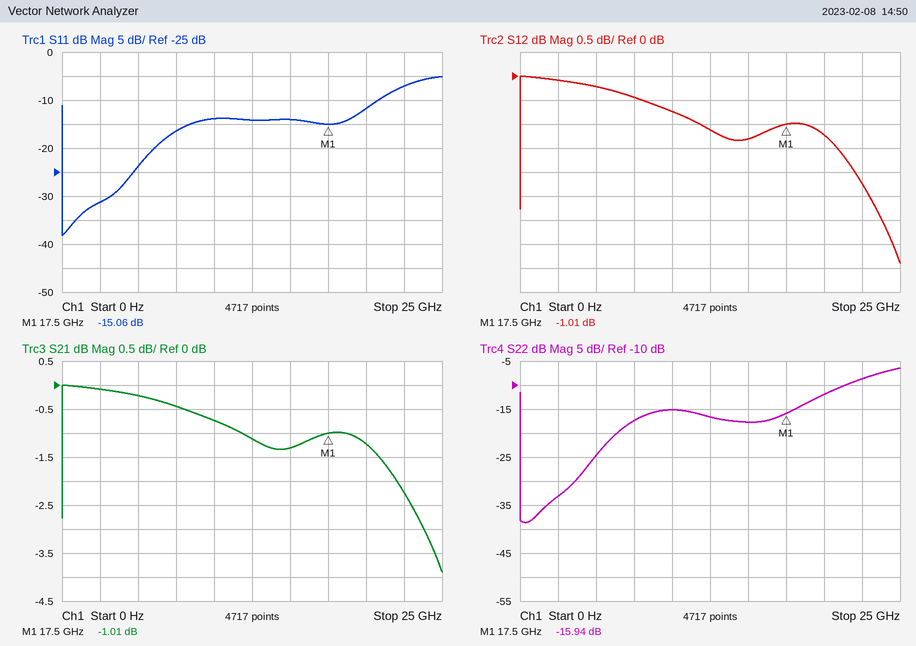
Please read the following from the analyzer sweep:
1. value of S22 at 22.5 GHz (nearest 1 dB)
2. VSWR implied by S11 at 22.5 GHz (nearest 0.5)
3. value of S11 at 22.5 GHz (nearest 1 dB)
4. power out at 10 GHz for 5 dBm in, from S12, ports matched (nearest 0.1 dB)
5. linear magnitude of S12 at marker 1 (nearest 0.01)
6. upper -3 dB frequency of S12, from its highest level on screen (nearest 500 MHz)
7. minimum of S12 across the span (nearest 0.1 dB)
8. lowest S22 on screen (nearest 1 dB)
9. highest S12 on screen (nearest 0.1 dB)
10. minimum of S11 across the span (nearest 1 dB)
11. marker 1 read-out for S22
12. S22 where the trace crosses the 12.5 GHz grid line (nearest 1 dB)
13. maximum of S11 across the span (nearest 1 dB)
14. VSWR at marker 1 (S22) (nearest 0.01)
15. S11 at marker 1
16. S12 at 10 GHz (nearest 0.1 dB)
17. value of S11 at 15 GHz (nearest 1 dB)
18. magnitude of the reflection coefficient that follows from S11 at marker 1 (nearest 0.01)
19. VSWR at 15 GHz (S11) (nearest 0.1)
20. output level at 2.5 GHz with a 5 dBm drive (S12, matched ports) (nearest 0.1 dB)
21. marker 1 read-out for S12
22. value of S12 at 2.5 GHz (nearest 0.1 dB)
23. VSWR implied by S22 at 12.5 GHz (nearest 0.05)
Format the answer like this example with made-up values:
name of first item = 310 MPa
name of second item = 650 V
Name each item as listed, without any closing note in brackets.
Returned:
value of S22 at 22.5 GHz = -9 dB
VSWR implied by S11 at 22.5 GHz = 2.5
value of S11 at 22.5 GHz = -7 dB
power out at 10 GHz for 5 dBm in, from S12, ports matched = 4.3 dBm
linear magnitude of S12 at marker 1 = 0.89
upper -3 dB frequency of S12, from its highest level on screen = 24.0 GHz
minimum of S12 across the span = -3.9 dB
lowest S22 on screen = -39 dB
highest S12 on screen = 0.0 dB
minimum of S11 across the span = -38 dB
marker 1 read-out for S22 = -15.94 dB
S22 where the trace crosses the 12.5 GHz grid line = -17 dB
maximum of S11 across the span = -5 dB
VSWR at marker 1 (S22) = 1.38
S11 at marker 1 = -15.06 dB
S12 at 10 GHz = -0.7 dB
value of S11 at 15 GHz = -14 dB
magnitude of the reflection coefficient that follows from S11 at marker 1 = 0.18
VSWR at 15 GHz (S11) = 1.5
output level at 2.5 GHz with a 5 dBm drive (S12, matched ports) = 4.9 dBm
marker 1 read-out for S12 = -1.01 dB
value of S12 at 2.5 GHz = -0.1 dB
VSWR implied by S22 at 12.5 GHz = 1.35
